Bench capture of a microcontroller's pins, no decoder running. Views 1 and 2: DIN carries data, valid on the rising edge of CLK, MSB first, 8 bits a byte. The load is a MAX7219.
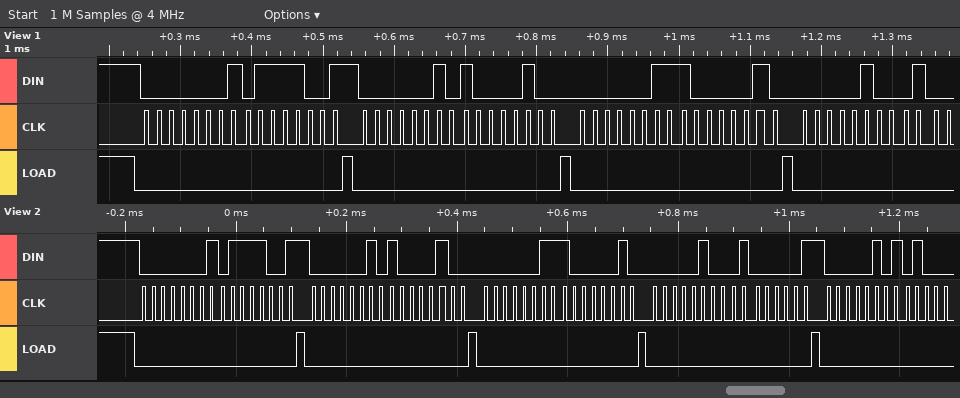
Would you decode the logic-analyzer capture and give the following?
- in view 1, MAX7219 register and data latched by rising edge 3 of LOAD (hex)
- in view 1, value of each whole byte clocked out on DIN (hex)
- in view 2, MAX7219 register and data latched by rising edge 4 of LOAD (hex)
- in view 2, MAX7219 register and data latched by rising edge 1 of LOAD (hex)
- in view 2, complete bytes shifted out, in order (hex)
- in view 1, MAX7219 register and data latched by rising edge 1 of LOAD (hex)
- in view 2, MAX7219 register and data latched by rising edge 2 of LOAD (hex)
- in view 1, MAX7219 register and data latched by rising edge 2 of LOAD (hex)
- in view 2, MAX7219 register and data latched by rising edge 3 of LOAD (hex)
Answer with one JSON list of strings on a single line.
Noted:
["register 0x3, data 0x82", "01 79 02 84 03 82 04", "register 0x4, data 0x41", "register 0x1, data 0x79", "0x01 0x79 0x02 0x84 0x03 0x82 0x04 0x41 0x05", "register 0x1, data 0x79", "register 0x2, data 0x84", "register 0x2, data 0x84", "register 0x3, data 0x82"]
